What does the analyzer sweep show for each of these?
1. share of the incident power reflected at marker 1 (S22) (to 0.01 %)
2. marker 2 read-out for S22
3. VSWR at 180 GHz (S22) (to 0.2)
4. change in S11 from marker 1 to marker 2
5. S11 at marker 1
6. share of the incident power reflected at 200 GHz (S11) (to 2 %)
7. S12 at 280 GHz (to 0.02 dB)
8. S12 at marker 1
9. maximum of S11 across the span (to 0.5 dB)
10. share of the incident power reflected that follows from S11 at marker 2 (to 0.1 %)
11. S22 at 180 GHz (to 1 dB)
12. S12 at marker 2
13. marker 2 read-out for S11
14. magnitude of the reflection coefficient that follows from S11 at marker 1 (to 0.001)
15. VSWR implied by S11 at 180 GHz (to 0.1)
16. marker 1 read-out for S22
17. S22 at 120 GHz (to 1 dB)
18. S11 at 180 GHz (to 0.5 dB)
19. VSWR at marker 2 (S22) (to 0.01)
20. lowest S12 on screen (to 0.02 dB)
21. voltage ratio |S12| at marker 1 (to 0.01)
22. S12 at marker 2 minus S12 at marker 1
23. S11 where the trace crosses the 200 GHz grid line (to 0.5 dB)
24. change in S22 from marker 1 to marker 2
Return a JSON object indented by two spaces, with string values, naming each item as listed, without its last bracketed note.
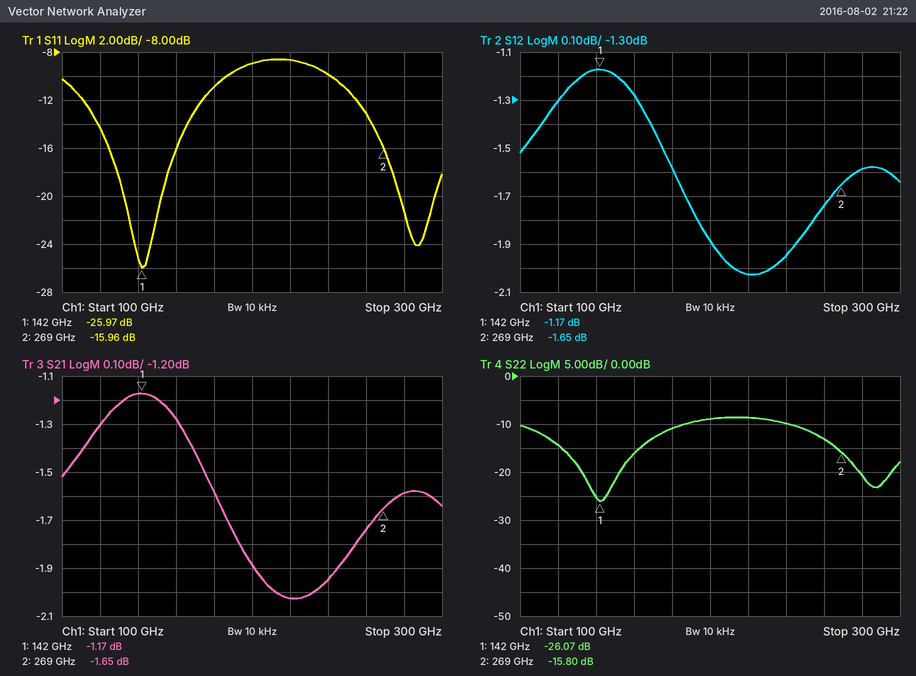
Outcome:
{
  "share of the incident power reflected at marker 1 (S22)": "0.25 %",
  "marker 2 read-out for S22": "-15.80 dB",
  "VSWR at 180 GHz (S22)": "1.8",
  "change in S11 from marker 1 to marker 2": "10.01 dB",
  "S11 at marker 1": "-25.97 dB",
  "share of the incident power reflected at 200 GHz (S11)": "12 %",
  "S12 at 280 GHz": "-1.58 dB",
  "S12 at marker 1": "-1.17 dB",
  "maximum of S11 across the span": "-8.5 dB",
  "share of the incident power reflected that follows from S11 at marker 2": "2.5 %",
  "S22 at 180 GHz": "-11 dB",
  "S12 at marker 2": "-1.65 dB",
  "marker 2 read-out for S11": "-15.96 dB",
  "magnitude of the reflection coefficient that follows from S11 at marker 1": "0.050",
  "VSWR implied by S11 at 180 GHz": "1.8",
  "marker 1 read-out for S22": "-26.07 dB",
  "S22 at 120 GHz": "-14 dB",
  "S11 at 180 GHz": "-11.0 dB",
  "VSWR at marker 2 (S22)": "1.39",
  "lowest S12 on screen": "-2.02 dB",
  "voltage ratio |S12| at marker 1": "0.87",
  "S12 at marker 2 minus S12 at marker 1": "-0.48 dB",
  "S11 where the trace crosses the 200 GHz grid line": "-9.0 dB",
  "change in S22 from marker 1 to marker 2": "10.27 dB"
}
